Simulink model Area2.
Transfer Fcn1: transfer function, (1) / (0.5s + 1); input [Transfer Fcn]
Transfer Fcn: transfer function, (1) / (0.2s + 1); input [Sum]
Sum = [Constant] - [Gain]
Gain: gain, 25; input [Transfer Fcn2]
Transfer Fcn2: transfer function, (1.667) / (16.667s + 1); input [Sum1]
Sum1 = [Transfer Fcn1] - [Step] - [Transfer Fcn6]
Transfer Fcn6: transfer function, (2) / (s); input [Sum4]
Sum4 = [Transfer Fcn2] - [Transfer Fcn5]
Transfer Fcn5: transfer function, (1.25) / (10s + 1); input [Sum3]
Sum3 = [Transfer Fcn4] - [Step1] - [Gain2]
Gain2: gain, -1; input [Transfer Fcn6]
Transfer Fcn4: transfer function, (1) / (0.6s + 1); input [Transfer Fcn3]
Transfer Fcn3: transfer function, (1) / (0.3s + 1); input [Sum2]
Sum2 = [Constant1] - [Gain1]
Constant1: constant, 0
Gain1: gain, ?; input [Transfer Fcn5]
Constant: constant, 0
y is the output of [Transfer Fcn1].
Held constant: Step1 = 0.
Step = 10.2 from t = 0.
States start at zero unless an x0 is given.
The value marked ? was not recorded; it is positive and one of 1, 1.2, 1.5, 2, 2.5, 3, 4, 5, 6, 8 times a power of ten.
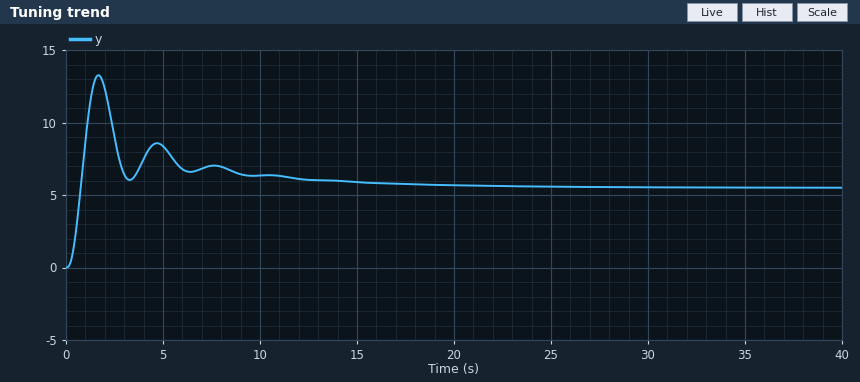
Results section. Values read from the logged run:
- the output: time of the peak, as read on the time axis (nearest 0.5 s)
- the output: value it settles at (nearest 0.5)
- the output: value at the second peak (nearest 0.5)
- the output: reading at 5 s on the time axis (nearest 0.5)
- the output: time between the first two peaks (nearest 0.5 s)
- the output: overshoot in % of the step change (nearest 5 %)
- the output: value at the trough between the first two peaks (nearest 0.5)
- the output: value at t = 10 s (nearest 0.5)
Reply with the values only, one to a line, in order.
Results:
1.5 s
5.5
8.5
8.5
3.0 s
140 %
6.0
6.5
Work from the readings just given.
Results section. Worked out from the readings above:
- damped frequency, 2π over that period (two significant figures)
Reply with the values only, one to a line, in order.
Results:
2.1 rad/s
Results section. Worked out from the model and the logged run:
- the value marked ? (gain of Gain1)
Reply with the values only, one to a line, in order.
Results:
20
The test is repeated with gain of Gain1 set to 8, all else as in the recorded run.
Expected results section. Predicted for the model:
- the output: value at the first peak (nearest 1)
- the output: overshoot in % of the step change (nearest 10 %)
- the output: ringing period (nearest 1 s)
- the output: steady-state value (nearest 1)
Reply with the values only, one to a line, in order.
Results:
13
80 %
3 s
7
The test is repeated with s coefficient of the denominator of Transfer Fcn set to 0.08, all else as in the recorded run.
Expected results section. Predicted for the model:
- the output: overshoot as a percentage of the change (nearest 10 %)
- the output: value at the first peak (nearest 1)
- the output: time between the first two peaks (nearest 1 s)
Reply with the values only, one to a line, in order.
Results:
120 %
12
3 s
